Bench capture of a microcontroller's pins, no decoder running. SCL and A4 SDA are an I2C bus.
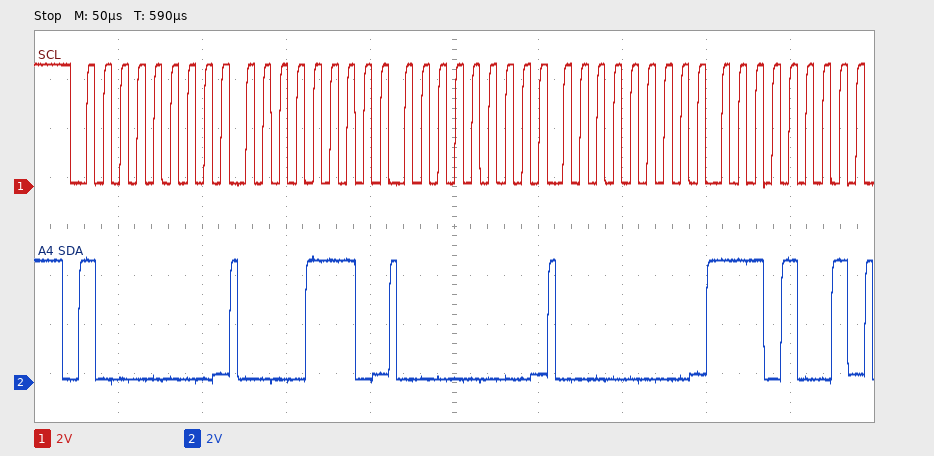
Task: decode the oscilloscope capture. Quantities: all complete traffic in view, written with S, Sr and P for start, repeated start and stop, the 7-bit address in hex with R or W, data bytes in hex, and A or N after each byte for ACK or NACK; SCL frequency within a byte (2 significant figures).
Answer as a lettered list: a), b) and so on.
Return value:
a) S 40W A 0E A 00 A 00 A E9 A
b) 100 kHz
